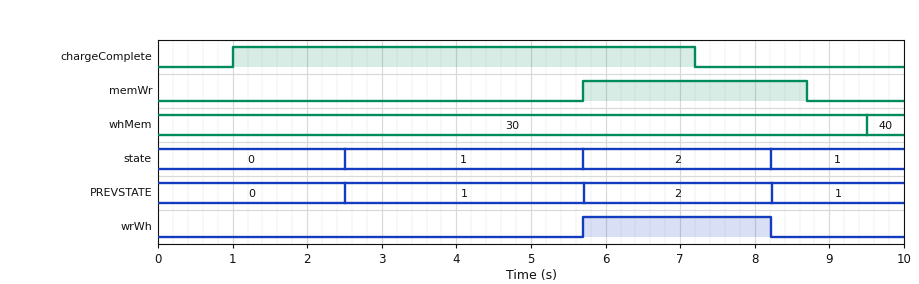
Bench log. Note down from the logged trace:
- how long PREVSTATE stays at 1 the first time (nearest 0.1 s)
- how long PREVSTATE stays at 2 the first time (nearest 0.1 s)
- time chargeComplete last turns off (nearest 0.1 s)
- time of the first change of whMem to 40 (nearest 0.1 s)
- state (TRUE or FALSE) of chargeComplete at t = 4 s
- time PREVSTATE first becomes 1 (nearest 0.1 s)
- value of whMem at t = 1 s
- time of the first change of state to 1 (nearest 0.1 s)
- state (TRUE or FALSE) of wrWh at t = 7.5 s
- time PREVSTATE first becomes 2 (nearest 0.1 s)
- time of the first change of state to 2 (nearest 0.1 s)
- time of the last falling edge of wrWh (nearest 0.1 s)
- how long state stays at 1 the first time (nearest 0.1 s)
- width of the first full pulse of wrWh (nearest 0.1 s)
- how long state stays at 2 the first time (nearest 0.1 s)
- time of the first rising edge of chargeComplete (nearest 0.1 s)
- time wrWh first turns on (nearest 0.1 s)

3.2 s
2.5 s
7.2 s
9.5 s
TRUE
2.5 s
30
2.5 s
TRUE
5.7 s
5.7 s
8.2 s
3.2 s
2.5 s
2.5 s
1.0 s
5.7 s
